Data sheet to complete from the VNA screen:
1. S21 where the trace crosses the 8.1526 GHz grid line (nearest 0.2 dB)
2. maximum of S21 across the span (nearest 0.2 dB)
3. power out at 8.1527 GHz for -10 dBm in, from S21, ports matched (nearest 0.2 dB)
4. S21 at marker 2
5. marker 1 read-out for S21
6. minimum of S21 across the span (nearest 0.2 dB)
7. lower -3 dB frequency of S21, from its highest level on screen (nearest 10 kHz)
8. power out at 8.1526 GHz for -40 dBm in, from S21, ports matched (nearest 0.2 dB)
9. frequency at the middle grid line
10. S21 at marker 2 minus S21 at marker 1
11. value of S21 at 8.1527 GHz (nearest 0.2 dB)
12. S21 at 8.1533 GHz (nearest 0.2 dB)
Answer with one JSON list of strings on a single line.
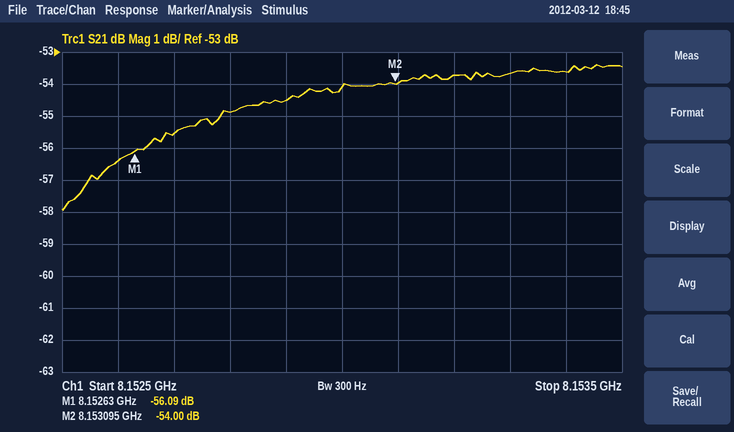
["-56.4 dB", "-53.4 dB", "-65.6 dBm", "-54.00 dB", "-56.09 dB", "-58.0 dB", "8.15260 GHz", "-96.4 dBm", "8.153 GHz", "2.09 dB", "-55.6 dB", "-53.6 dB"]
